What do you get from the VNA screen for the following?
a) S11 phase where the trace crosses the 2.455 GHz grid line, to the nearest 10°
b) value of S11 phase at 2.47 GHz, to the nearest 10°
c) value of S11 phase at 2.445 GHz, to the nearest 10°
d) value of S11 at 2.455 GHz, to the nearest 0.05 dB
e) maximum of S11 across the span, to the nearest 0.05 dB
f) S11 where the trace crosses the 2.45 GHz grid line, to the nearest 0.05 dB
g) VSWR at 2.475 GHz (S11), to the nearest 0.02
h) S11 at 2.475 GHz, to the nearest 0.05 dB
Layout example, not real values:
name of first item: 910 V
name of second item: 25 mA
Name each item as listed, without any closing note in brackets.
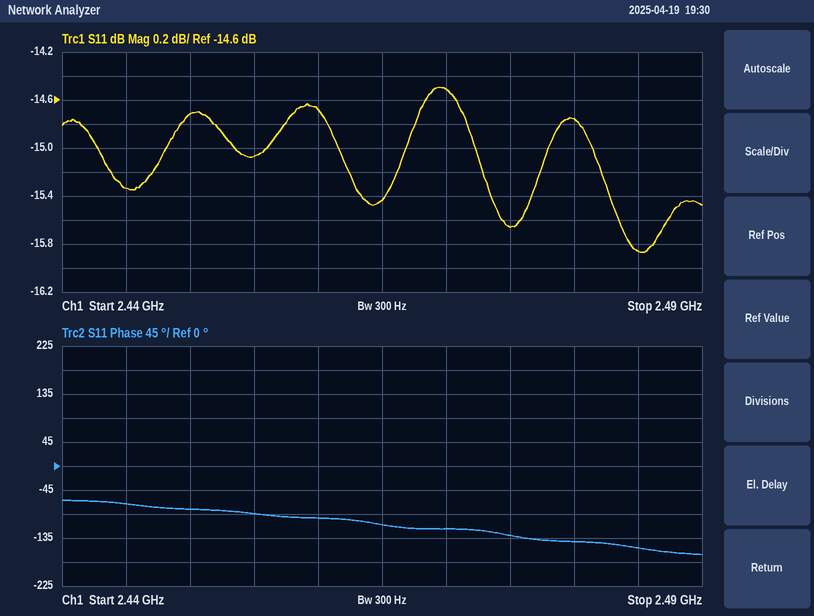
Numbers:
S11 phase where the trace crosses the 2.455 GHz grid line, to the nearest 10°: -90°
value of S11 phase at 2.47 GHz, to the nearest 10°: -120°
value of S11 phase at 2.445 GHz, to the nearest 10°: -70°
value of S11 at 2.455 GHz, to the nearest 0.05 dB: -15.05 dB
maximum of S11 across the span, to the nearest 0.05 dB: -14.50 dB
S11 where the trace crosses the 2.45 GHz grid line, to the nearest 0.05 dB: -14.70 dB
VSWR at 2.475 GHz (S11), to the nearest 0.02: 1.40
S11 at 2.475 GHz, to the nearest 0.05 dB: -15.65 dB
